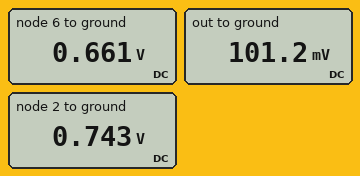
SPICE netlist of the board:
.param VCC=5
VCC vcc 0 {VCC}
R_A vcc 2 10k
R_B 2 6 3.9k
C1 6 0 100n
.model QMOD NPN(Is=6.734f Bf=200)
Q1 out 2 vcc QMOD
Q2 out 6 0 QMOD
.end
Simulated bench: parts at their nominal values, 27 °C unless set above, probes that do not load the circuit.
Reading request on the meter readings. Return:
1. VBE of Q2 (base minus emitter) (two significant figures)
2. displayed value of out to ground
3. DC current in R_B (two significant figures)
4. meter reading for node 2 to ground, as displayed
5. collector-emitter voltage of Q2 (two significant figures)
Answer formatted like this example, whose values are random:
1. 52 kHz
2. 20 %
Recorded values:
1. 660 mV
2. 101.2 mV
3. 21 µA
4. 0.743 V
5. 100 mV
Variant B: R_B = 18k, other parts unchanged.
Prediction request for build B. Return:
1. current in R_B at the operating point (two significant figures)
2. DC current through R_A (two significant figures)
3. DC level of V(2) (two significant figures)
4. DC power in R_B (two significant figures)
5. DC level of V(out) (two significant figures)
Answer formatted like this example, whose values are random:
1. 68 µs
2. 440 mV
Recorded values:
1. 7.1 µA
2. 420 µA
3. 790 mV
4. 910 nW
5. 150 mV
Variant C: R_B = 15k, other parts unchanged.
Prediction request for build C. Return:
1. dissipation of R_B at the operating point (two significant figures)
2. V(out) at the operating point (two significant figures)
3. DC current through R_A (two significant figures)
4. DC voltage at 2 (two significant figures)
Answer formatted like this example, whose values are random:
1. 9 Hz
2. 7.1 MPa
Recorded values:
1. 970 nW
2. 140 mV
3. 420 µA
4. 780 mV
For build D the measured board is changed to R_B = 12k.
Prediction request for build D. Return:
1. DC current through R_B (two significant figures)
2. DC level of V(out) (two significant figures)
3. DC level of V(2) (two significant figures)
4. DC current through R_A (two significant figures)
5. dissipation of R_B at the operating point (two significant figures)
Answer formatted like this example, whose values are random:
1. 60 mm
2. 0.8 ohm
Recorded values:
1. 9.4 µA
2. 130 mV
3. 770 mV
4. 420 µA
5. 1.1 µW
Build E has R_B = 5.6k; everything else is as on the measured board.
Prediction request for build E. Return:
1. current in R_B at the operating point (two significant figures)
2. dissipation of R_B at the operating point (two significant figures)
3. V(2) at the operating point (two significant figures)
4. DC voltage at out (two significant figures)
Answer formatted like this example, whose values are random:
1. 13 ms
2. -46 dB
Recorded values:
1. 16 µA
2. 1.5 µW
3. 750 mV
4. 110 mV
